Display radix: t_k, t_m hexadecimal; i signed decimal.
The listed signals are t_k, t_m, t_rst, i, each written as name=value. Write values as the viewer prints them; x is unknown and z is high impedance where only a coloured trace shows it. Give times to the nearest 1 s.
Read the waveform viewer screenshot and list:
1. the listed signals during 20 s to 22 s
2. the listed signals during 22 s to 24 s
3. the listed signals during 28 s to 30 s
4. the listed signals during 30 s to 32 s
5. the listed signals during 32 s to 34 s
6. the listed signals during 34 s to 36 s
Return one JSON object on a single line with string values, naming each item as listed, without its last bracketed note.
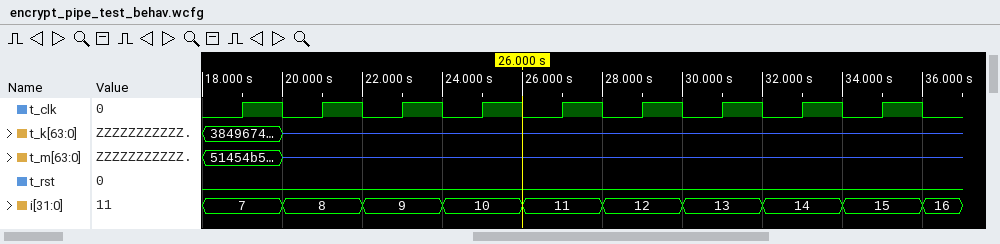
{"the listed signals during 20 s to 22 s": "t_k=z, t_m=z, t_rst=0, i=8", "the listed signals during 22 s to 24 s": "t_k=z, t_m=z, t_rst=0, i=9", "the listed signals during 28 s to 30 s": "t_k=z, t_m=z, t_rst=0, i=12", "the listed signals during 30 s to 32 s": "t_k=z, t_m=z, t_rst=0, i=13", "the listed signals during 32 s to 34 s": "t_k=z, t_m=z, t_rst=0, i=14", "the listed signals during 34 s to 36 s": "t_k=z, t_m=z, t_rst=0, i=15"}
